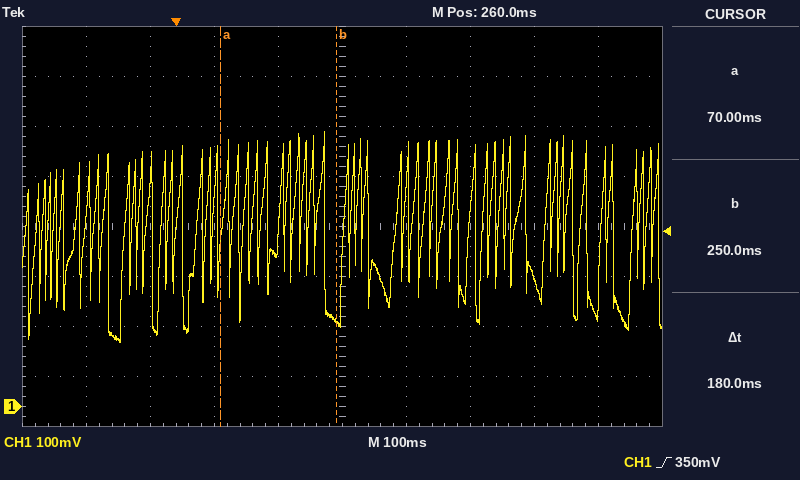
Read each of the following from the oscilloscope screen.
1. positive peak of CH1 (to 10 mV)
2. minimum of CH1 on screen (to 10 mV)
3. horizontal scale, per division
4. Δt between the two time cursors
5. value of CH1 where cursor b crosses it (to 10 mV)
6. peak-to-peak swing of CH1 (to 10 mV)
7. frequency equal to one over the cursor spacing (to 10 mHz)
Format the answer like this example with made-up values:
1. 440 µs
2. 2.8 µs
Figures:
1. 550 mV
2. 130 mV
3. 100 ms
4. 180 ms
5. 170 mV
6. 420 mV
7. 5.56 Hz
